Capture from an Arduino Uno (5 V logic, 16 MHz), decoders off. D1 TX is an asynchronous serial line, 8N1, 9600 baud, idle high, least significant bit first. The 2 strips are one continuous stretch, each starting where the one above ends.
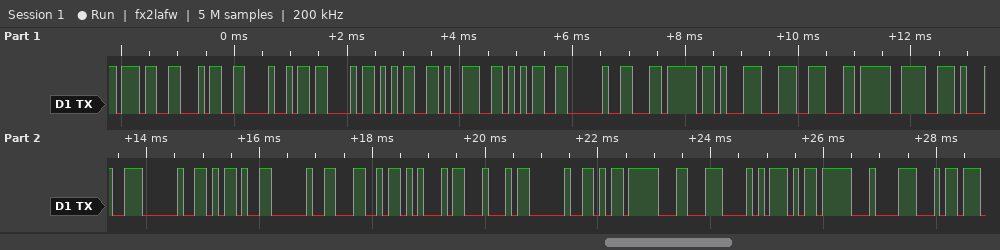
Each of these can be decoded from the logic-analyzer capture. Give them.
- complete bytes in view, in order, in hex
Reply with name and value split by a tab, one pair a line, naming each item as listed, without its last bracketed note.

complete bytes in view, in order, in hex	0x37 0x34 0x48 0x43 0x35 0x39 0x35 0x20 0xEC 0x8B 0x9C 0xEC 0x9E 0x91 0x20 0x2D 0x20 0x4C 0x45 0x44 0x20 0xED 0x8C 0xA8 0xED 0x84 0xB4
